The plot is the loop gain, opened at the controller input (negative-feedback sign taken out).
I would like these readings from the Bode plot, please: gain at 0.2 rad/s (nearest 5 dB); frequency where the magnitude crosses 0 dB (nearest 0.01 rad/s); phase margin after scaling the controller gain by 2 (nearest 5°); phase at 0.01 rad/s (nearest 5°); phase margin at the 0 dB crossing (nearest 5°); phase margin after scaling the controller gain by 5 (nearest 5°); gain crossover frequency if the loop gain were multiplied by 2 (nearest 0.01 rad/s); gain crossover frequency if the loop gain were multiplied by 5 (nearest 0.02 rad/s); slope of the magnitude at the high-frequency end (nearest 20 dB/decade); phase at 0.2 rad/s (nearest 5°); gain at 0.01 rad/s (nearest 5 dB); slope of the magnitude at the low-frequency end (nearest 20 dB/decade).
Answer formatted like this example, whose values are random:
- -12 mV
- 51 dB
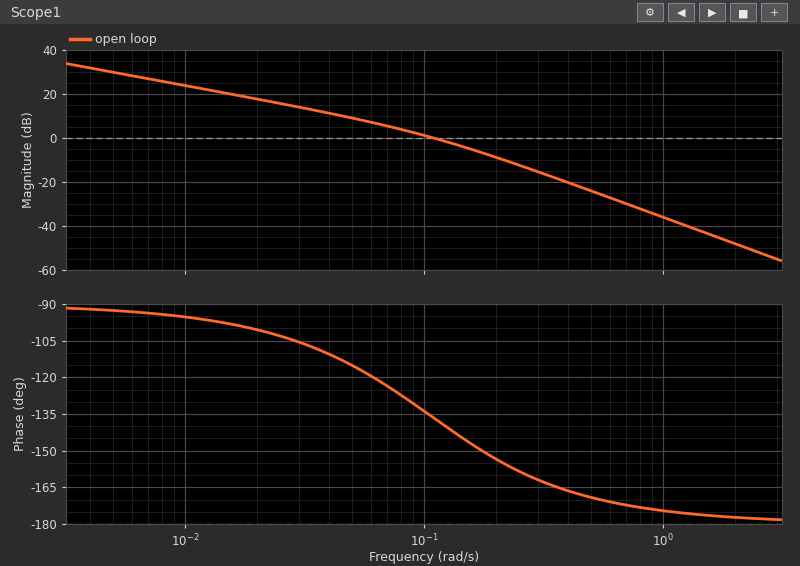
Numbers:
- -10 dB
- 0.11 rad/s
- 30°
- -95°
- 45°
- 20°
- 0.17 rad/s
- 0.28 rad/s
- -40 dB/decade
- -155°
- 25 dB
- -20 dB/decade
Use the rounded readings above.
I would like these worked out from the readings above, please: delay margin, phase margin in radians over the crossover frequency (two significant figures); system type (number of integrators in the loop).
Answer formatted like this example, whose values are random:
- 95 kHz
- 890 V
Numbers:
- 7.1 s
- 1
